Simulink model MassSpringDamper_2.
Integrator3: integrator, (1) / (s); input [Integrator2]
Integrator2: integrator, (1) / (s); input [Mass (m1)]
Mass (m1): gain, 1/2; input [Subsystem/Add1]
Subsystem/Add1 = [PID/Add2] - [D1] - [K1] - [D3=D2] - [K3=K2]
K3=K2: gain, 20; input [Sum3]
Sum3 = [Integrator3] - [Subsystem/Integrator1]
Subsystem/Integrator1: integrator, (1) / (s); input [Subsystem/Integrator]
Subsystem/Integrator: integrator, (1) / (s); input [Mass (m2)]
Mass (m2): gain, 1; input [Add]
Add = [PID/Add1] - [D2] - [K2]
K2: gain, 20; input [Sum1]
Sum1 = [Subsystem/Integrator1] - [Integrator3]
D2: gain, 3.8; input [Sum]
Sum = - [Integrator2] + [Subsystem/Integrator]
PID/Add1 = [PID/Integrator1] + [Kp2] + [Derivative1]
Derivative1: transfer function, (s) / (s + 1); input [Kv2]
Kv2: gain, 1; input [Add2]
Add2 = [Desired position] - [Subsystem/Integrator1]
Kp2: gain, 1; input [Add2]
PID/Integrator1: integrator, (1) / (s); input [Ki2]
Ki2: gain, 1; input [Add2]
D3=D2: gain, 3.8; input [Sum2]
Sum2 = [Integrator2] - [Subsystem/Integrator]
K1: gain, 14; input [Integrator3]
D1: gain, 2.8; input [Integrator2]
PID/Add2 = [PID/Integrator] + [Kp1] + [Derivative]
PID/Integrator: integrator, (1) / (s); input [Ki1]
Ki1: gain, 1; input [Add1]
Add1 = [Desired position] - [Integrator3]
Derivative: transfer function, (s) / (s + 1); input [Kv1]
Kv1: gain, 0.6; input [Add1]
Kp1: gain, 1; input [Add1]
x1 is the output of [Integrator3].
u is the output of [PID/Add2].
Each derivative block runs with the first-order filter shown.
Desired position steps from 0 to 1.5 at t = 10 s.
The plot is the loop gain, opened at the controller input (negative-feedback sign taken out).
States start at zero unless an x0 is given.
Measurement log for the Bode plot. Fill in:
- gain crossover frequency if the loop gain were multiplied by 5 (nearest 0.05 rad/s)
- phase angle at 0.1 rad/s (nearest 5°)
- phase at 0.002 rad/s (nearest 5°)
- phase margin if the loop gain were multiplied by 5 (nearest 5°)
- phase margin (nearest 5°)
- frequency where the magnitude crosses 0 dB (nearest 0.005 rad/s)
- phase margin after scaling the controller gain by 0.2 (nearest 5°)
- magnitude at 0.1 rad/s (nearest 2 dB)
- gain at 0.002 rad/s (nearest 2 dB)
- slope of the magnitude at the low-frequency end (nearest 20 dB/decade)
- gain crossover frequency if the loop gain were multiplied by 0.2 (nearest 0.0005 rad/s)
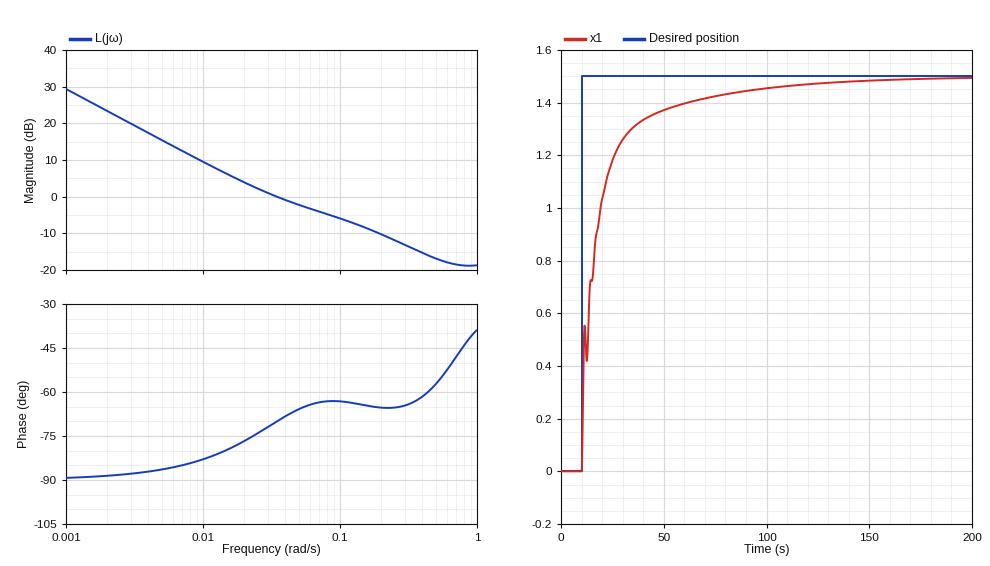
0.35 rad/s
-65°
-90°
115°
110°
0.035 rad/s
95°
-6 dB
24 dB
-20 dB/decade
0.0060 rad/s
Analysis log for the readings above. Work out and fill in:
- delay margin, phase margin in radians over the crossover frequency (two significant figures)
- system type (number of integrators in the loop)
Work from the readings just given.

55 s
1
